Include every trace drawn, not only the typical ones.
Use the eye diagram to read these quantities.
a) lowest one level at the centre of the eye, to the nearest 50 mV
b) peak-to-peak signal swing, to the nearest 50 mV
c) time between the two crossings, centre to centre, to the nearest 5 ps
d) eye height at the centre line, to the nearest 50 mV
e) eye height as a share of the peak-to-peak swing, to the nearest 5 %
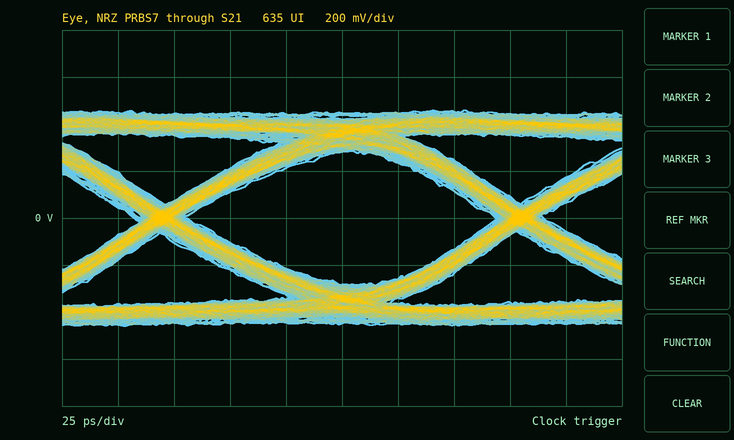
300 mV
900 mV
160 ps
550 mV
60 %
